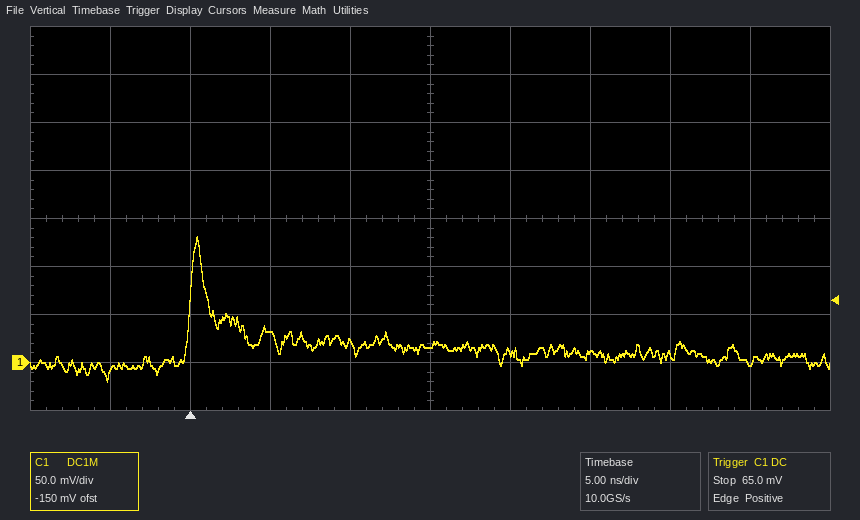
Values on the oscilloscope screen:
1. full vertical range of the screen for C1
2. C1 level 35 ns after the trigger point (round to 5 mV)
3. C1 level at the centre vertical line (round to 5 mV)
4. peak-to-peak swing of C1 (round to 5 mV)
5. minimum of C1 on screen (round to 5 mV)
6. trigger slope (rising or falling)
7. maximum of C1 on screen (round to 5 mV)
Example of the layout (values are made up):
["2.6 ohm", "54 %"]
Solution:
["400 mV", "0 mV", "20 mV", "150 mV", "-20 mV", "rising", "130 mV"]
